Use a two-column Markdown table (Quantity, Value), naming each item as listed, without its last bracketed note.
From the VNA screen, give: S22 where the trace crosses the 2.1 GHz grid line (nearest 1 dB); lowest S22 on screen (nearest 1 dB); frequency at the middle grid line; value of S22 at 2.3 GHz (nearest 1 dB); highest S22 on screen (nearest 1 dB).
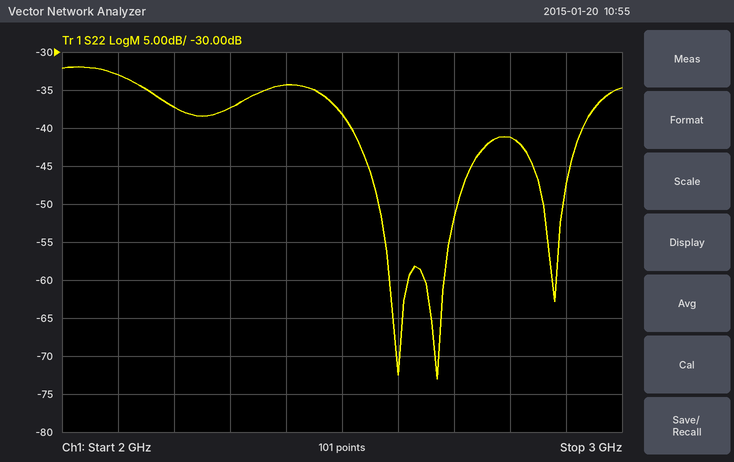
| Quantity | Value |
|---|---|
| S22 where the trace crosses the 2.1 GHz grid line | -33 dB |
| lowest S22 on screen | -73 dB |
| frequency at the middle grid line | 2.5 GHz |
| value of S22 at 2.3 GHz | -37 dB |
| highest S22 on screen | -32 dB |
